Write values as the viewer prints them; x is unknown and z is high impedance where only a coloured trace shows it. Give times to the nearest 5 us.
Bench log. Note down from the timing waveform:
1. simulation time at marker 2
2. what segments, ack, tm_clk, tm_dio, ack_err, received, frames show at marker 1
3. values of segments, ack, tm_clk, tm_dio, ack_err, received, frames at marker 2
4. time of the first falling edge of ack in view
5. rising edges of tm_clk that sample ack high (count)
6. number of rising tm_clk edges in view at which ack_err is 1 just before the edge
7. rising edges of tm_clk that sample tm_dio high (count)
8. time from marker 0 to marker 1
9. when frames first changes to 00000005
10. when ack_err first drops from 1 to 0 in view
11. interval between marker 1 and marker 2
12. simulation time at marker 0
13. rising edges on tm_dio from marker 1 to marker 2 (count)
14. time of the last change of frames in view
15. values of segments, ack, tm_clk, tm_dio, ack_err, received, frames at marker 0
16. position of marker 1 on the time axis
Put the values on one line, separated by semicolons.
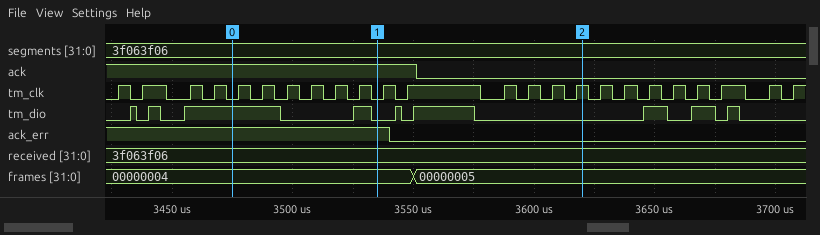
3620 us; segments=3f063f06, ack=1, tm_clk=0, tm_dio=0, ack_err=1, received=3f063f06, frames=00000004; segments=3f063f06, ack=0, tm_clk=1, tm_dio=0, ack_err=0, received=3f063f06, frames=00000005; 3550 us; 12; 11; 7; 60 us; 3550 us; 3540 us; 85 us; 3475 us; 2; 3550 us; segments=3f063f06, ack=1, tm_clk=0, tm_dio=1, ack_err=1, received=3f063f06, frames=00000004; 3535 us
